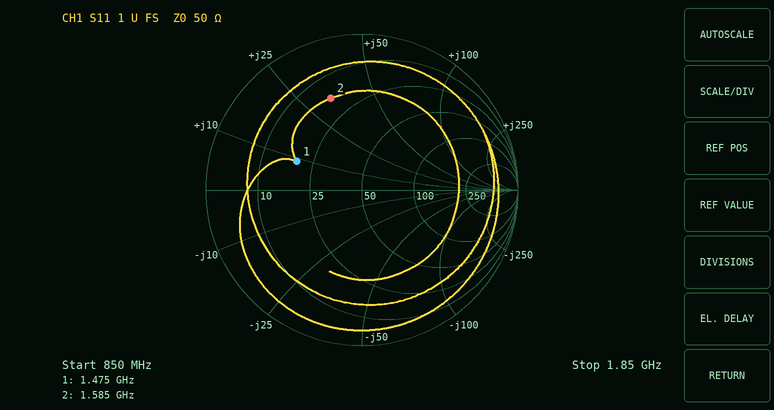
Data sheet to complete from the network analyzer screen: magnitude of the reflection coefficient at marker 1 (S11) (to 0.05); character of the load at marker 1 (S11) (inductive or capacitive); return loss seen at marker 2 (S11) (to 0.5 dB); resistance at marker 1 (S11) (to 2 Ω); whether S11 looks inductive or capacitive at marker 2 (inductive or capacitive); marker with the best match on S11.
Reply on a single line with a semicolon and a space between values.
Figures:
0.45; inductive; 4.0 dB; 20 Ω; inductive; marker 1
